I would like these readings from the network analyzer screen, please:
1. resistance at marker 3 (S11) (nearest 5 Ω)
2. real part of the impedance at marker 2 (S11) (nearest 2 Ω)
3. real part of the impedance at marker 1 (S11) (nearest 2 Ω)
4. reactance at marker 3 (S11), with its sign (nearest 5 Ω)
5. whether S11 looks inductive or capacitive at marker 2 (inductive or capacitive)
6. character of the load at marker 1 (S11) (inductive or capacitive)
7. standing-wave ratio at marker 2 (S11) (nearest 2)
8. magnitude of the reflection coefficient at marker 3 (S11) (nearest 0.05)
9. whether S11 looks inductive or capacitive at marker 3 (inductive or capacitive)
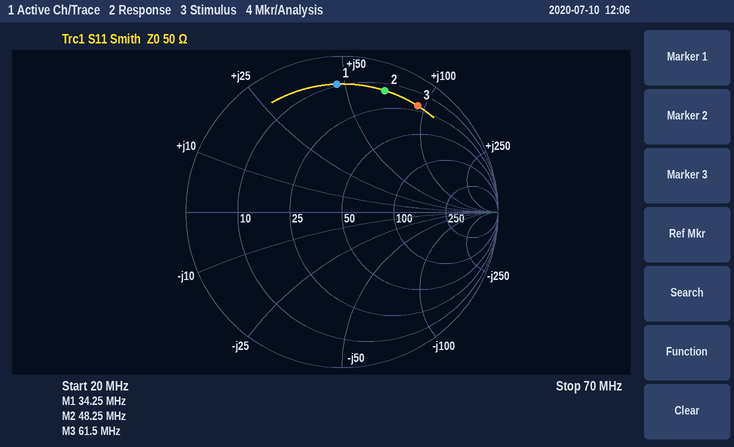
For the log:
20 Ω
14 Ω
10 Ω
+95 Ω
inductive
inductive
10
0.85
inductive
